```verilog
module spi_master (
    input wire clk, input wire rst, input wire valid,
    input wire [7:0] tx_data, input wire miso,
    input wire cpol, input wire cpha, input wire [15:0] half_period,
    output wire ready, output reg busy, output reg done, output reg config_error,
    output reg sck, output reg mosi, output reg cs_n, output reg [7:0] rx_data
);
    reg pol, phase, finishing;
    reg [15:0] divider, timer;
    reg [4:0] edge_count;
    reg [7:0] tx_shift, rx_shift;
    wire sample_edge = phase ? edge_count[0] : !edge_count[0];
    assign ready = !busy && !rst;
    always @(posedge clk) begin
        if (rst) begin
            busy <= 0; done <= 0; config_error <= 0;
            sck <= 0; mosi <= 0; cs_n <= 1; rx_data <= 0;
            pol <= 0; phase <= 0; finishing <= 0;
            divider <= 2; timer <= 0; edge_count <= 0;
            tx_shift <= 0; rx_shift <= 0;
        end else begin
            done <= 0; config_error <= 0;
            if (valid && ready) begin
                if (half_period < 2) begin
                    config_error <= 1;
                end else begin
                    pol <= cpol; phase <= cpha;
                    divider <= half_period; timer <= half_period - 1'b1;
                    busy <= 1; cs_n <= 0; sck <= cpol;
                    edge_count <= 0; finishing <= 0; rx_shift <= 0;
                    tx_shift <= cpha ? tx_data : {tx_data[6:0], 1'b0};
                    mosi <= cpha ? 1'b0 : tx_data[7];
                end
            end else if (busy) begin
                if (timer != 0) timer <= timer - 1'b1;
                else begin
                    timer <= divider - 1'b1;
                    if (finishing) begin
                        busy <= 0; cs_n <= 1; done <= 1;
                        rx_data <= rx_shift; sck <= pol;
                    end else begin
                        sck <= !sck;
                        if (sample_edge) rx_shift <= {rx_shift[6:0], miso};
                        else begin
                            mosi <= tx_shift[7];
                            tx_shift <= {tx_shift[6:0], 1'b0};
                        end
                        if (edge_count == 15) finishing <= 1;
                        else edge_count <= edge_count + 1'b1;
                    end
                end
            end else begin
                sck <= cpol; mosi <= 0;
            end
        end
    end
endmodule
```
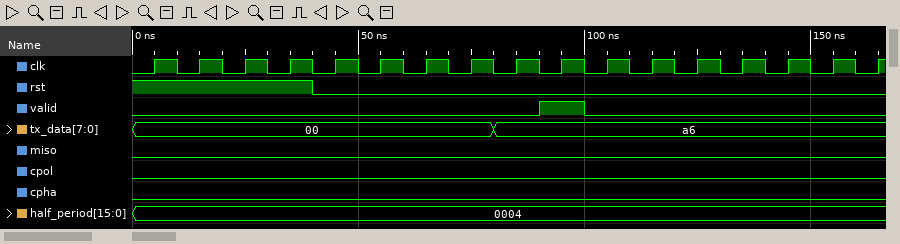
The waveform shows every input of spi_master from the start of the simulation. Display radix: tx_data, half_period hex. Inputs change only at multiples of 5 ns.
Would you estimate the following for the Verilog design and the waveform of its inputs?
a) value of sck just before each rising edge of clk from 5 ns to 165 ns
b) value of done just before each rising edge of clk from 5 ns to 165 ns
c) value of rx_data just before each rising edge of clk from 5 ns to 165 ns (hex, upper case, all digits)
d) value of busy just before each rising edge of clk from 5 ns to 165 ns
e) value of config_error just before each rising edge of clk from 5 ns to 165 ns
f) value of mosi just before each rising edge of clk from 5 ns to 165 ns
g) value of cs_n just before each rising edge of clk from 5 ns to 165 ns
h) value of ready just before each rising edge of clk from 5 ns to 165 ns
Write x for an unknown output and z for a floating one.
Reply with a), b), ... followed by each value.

a) x 0 0 0 0 0 0 0 0 0 0 0 0 0 1 1 1
b) x 0 0 0 0 0 0 0 0 0 0 0 0 0 0 0 0
c) x, 00, 00, 00, 00, 00, 00, 00, 00, 00, 00, 00, 00, 00, 00, 00, 00
d) x 0 0 0 0 0 0 0 0 0 1 1 1 1 1 1 1
e) x 0 0 0 0 0 0 0 0 0 0 0 0 0 0 0 0
f) x 0 0 0 0 0 0 0 0 0 1 1 1 1 1 1 1
g) x 1 1 1 1 1 1 1 1 1 0 0 0 0 0 0 0
h) 0 0 0 0 1 1 1 1 1 1 0 0 0 0 0 0 0
